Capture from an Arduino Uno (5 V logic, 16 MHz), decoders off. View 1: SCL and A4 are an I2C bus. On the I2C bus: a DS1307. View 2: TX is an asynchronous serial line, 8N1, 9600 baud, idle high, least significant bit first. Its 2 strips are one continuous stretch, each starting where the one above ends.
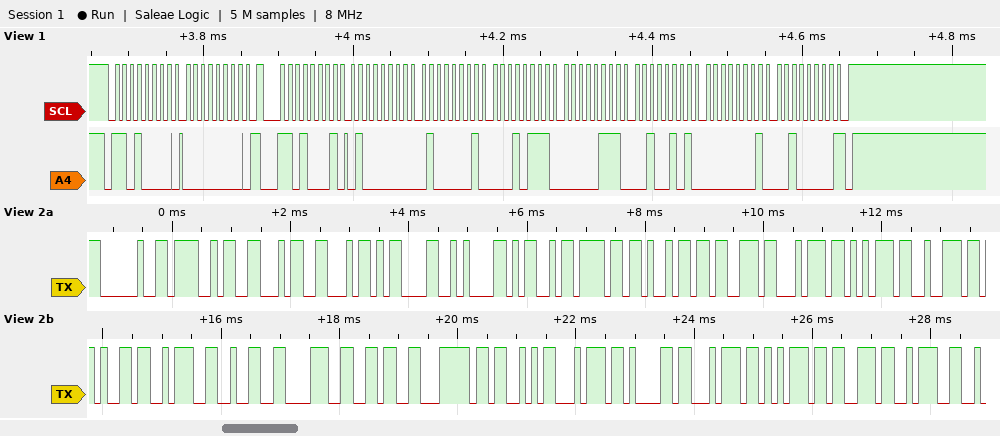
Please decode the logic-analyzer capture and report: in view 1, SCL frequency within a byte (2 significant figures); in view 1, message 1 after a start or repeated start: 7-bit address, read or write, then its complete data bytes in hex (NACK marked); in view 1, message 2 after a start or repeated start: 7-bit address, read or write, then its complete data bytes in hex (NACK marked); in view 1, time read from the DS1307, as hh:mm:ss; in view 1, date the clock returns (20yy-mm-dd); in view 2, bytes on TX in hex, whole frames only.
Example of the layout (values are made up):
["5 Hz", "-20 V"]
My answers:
["100 kHz", "0x68 write: 00", "0x68 read: 40 41 17 07 25 01 20 NACK", "17:41:40", "2020-01-25", "20 4F 46 46 0D 0A 4D 6F 69 73 74 75 72 65 3A 32 38 36 7C 53 74 61 74 75 73 3A"]
